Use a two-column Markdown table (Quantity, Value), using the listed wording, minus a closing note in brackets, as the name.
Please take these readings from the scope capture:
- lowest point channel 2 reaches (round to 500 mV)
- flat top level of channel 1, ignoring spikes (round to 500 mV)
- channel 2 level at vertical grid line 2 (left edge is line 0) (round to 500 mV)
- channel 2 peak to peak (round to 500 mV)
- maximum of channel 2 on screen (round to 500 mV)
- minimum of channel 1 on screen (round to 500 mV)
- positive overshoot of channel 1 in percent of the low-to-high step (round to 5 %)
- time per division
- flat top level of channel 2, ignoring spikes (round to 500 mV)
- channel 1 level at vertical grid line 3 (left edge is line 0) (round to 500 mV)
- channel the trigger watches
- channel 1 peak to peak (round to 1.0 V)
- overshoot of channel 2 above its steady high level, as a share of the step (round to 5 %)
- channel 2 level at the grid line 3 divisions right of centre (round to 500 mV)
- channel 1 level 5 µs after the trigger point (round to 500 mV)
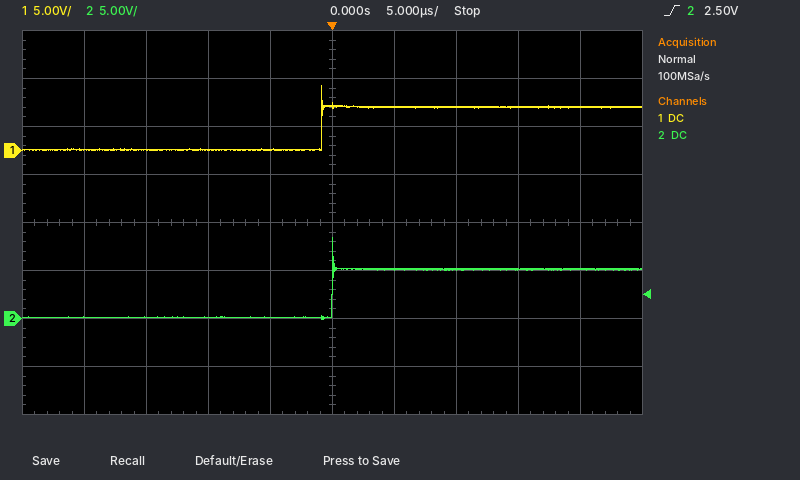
| Quantity | Value |
|---|---|
| lowest point channel 2 reaches | 0.0 V |
| flat top level of channel 1, ignoring spikes | 4.5 V |
| channel 2 level at vertical grid line 2 (left edge is line 0) | 0.0 V |
| channel 2 peak to peak | 8.5 V |
| maximum of channel 2 on screen | 8.5 V |
| minimum of channel 1 on screen | 0.0 V |
| positive overshoot of channel 1 in percent of the low-to-high step | 50 % |
| time per division | 5 µs |
| flat top level of channel 2, ignoring spikes | 5.0 V |
| channel 1 level at vertical grid line 3 (left edge is line 0) | 0.0 V |
| channel the trigger watches | channel 2 |
| channel 1 peak to peak | 7.0 V |
| overshoot of channel 2 above its steady high level, as a share of the step | 65 % |
| channel 2 level at the grid line 3 divisions right of centre | 5.0 V |
| channel 1 level 5 µs after the trigger point | 4.5 V |
